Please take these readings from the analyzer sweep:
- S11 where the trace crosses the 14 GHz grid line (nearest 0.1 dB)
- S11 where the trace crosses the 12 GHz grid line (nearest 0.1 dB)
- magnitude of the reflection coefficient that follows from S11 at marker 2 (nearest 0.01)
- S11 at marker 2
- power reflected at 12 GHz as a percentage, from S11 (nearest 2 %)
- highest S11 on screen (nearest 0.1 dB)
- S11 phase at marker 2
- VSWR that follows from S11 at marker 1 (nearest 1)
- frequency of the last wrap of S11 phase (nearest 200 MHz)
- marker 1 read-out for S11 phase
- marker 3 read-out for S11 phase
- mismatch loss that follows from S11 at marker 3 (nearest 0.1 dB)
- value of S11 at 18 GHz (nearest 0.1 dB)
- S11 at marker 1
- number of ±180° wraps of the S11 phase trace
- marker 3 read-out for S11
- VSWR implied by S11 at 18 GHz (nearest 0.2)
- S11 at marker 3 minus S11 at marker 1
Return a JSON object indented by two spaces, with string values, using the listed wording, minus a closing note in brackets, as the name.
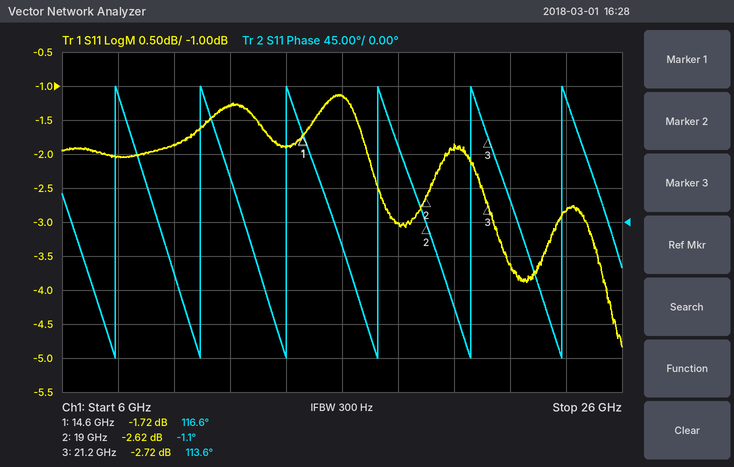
{
  "S11 where the trace crosses the 14 GHz grid line": "-1.9 dB",
  "S11 where the trace crosses the 12 GHz grid line": "-1.3 dB",
  "magnitude of the reflection coefficient that follows from S11 at marker 2": "0.74",
  "S11 at marker 2": "-2.62 dB",
  "power reflected at 12 GHz as a percentage, from S11": "74 %",
  "highest S11 on screen": "-1.1 dB",
  "S11 phase at marker 2": "-1.1°",
  "VSWR that follows from S11 at marker 1": "10",
  "frequency of the last wrap of S11 phase": "23.8 GHz",
  "marker 1 read-out for S11 phase": "116.6°",
  "marker 3 read-out for S11 phase": "113.6°",
  "mismatch loss that follows from S11 at marker 3": "3.3 dB",
  "value of S11 at 18 GHz": "-3.0 dB",
  "S11 at marker 1": "-1.72 dB",
  "number of ±180° wraps of the S11 phase trace": "6",
  "marker 3 read-out for S11": "-2.72 dB",
  "VSWR implied by S11 at 18 GHz": "5.8",
  "S11 at marker 3 minus S11 at marker 1": "-1.00 dB"
}
